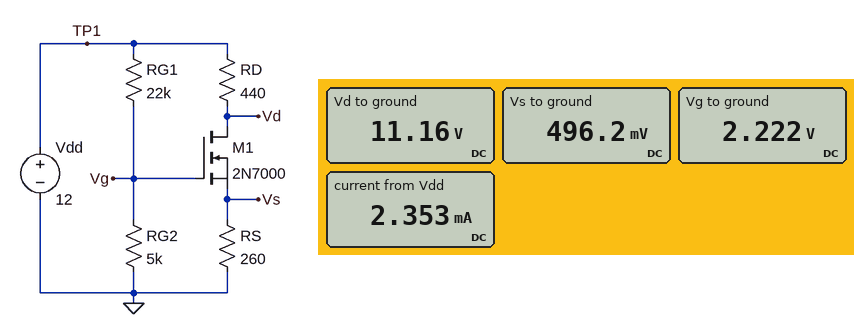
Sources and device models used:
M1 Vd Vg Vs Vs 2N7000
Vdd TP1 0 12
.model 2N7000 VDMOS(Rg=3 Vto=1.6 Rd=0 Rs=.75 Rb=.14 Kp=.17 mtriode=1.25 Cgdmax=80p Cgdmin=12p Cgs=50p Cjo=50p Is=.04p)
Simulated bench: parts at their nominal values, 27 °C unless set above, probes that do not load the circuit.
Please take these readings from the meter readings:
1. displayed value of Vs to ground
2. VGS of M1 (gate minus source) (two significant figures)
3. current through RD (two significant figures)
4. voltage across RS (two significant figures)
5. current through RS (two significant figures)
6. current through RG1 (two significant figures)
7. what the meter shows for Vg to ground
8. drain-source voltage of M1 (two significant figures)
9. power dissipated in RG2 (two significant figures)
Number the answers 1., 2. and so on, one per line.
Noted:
1. 496.2 mV
2. 1.7 V
3. 1.9 mA
4. 500 mV
5. 1.9 mA
6. 440 µA
7. 2.222 V
8. 11 V
9. 990 µW
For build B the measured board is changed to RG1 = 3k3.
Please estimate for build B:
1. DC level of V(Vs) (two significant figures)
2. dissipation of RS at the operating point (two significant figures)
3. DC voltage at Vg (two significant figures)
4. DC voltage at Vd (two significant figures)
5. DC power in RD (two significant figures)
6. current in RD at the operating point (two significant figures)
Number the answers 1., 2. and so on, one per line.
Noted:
1. 4.4 V
2. 75 mW
3. 7.2 V
4. 4.5 V
5. 130 mW
6. 17 mA
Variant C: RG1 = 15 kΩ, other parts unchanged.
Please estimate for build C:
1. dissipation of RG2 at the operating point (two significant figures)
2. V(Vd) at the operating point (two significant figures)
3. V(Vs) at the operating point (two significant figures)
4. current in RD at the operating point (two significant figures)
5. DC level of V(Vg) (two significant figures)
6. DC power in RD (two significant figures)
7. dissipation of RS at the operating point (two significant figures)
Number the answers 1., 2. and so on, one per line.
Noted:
1. 1.8 mW
2. 10 V
3. 1.2 V
4. 4.5 mA
5. 3.0 V
6. 9.0 mW
7. 5.3 mW
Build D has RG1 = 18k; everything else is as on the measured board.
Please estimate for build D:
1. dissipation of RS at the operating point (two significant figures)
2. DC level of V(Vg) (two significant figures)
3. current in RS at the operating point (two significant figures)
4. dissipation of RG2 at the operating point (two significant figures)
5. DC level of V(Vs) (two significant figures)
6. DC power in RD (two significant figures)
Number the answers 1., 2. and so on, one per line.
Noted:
1. 2.6 mW
2. 2.6 V
3. 3.2 mA
4. 1.4 mW
5. 830 mV
6. 4.5 mW
